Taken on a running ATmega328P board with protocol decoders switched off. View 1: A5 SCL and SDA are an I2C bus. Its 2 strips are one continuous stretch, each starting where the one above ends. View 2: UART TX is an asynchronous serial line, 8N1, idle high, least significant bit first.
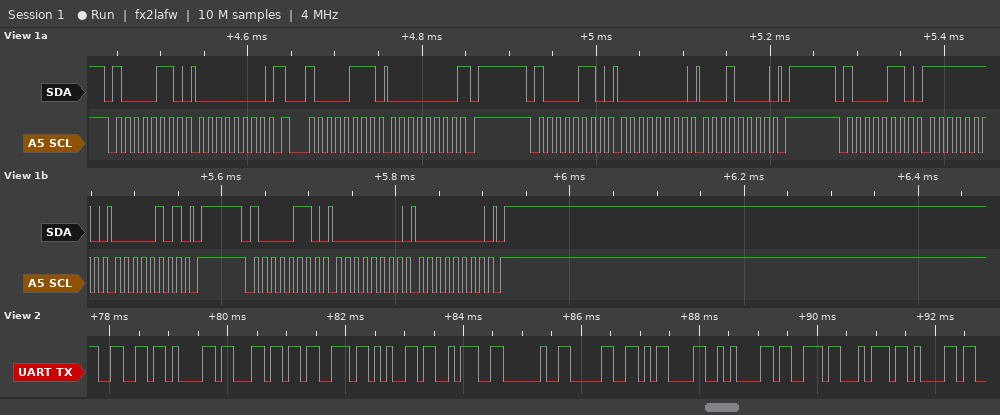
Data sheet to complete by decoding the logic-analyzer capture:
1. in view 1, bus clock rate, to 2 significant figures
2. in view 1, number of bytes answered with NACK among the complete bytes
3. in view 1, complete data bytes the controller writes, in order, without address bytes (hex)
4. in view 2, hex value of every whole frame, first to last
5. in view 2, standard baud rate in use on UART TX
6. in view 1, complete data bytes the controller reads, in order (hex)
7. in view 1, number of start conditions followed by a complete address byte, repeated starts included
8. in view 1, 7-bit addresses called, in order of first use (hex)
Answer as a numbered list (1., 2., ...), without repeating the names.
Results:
1. 100 kHz
2. 1
3. 00 00 10 FE 05 00 00
4. 66 61 6C 73 65 3A 20 30 0D 0A 73 74 61
5. 9600 baud
6. 00
7. 5
8. 0x43
